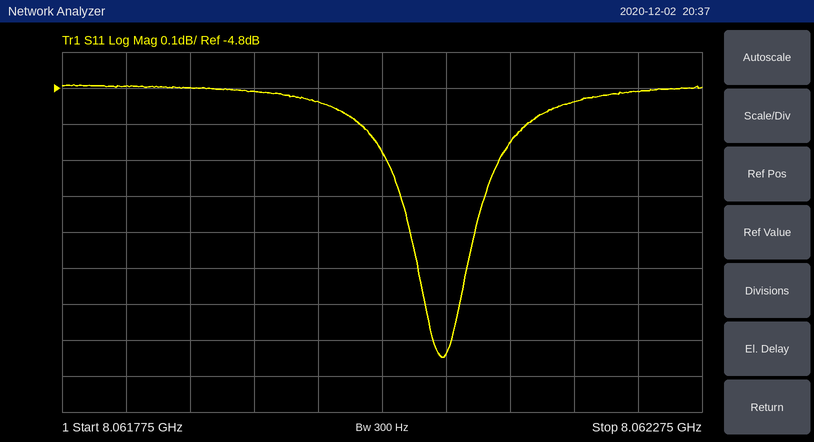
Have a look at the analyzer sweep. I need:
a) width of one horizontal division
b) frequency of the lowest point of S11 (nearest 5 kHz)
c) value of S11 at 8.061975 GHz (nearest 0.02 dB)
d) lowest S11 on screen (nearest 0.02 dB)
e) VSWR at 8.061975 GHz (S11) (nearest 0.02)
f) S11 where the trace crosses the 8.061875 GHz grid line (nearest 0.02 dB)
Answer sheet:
50 kHz
8.062070 GHz
-4.84 dB
-5.54 dB
3.68
-4.80 dB
